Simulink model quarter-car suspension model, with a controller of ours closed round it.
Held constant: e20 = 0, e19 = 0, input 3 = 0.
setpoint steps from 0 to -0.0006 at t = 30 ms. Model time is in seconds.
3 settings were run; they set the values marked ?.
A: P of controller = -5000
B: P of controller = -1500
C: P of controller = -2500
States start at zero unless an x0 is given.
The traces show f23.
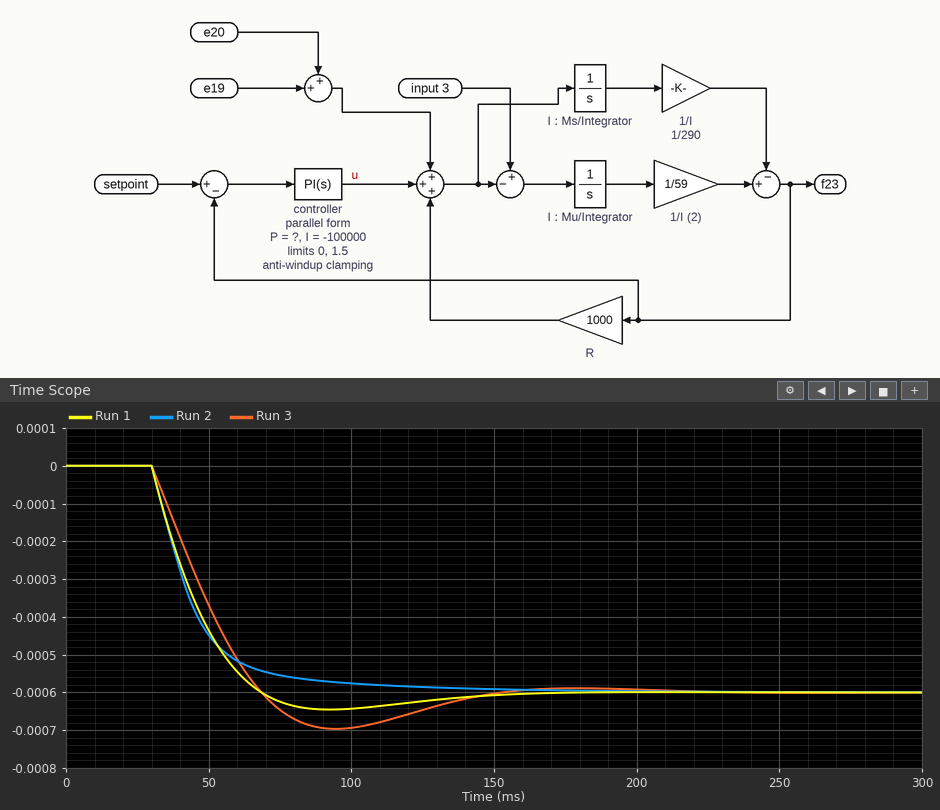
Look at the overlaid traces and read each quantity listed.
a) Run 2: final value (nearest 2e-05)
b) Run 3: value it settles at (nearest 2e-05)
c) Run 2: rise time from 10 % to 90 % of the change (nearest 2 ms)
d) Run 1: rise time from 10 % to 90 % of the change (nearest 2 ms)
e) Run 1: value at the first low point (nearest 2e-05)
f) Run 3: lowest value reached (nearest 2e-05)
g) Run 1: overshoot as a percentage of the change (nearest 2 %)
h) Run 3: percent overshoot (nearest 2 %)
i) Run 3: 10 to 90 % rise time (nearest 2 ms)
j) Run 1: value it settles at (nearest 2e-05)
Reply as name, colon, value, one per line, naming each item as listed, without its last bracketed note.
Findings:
Run 2: final value: -0.00060
Run 3: value it settles at: -0.00060
Run 2: rise time from 10 % to 90 % of the change: 36 ms
Run 1: rise time from 10 % to 90 % of the change: 28 ms
Run 1: value at the first low point: -0.00064
Run 3: lowest value reached: -0.00070
Run 1: overshoot as a percentage of the change: 8 %
Run 3: percent overshoot: 16 %
Run 3: 10 to 90 % rise time: 30 ms
Run 1: value it settles at: -0.00060
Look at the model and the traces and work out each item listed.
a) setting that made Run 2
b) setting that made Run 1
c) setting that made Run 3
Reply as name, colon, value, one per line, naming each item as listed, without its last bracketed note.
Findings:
setting that made Run 2: A
setting that made Run 1: C
setting that made Run 3: B
